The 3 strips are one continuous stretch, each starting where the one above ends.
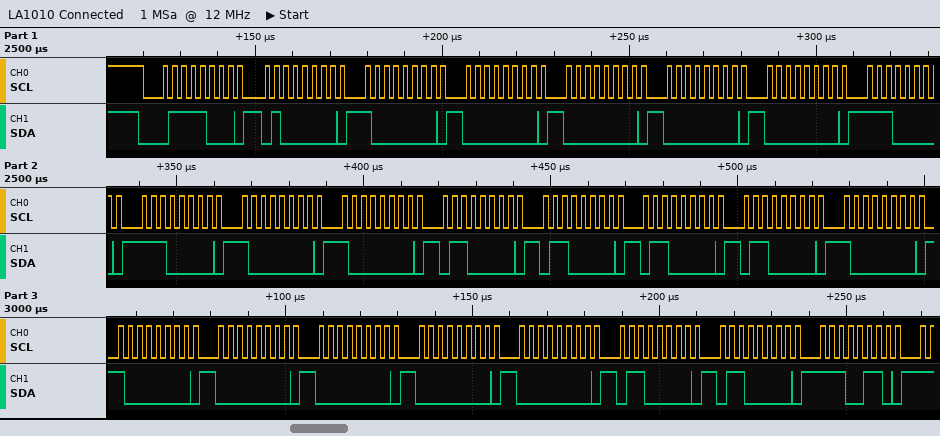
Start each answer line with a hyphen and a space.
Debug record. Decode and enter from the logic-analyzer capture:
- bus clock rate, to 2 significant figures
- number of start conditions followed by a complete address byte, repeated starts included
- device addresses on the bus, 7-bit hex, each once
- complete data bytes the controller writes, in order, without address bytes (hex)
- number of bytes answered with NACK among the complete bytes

- 400 kHz
- 1
- 0x3C
- 40 80 00 00 00 00 E0 E0 80 80 60 60 60 60 80 80 00 00 00 00 60 60 E6
- 0
